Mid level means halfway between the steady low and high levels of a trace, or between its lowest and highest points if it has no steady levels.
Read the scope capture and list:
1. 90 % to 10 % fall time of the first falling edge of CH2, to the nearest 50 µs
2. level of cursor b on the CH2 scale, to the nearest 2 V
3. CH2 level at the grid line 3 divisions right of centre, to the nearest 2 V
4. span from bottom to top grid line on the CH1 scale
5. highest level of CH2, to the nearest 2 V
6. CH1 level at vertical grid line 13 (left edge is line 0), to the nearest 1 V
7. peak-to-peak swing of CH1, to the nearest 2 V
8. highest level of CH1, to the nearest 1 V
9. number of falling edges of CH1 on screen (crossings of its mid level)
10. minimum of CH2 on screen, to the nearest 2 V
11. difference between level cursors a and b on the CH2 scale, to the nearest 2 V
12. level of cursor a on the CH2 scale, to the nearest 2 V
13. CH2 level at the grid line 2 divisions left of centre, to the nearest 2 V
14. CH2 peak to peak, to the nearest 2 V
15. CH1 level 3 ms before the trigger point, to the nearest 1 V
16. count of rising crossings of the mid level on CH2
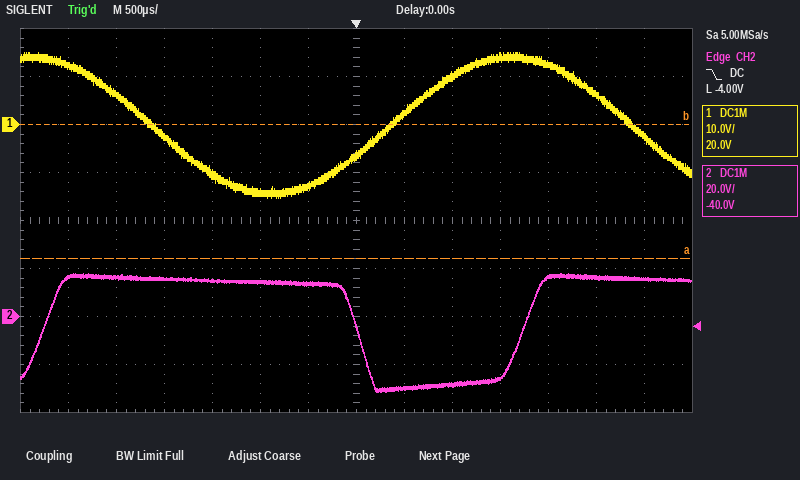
300 µs
80 V
-26 V
80 V
18 V
-2 V
30 V
15 V
2
-32 V
56 V
24 V
14 V
50 V
12 V
2
